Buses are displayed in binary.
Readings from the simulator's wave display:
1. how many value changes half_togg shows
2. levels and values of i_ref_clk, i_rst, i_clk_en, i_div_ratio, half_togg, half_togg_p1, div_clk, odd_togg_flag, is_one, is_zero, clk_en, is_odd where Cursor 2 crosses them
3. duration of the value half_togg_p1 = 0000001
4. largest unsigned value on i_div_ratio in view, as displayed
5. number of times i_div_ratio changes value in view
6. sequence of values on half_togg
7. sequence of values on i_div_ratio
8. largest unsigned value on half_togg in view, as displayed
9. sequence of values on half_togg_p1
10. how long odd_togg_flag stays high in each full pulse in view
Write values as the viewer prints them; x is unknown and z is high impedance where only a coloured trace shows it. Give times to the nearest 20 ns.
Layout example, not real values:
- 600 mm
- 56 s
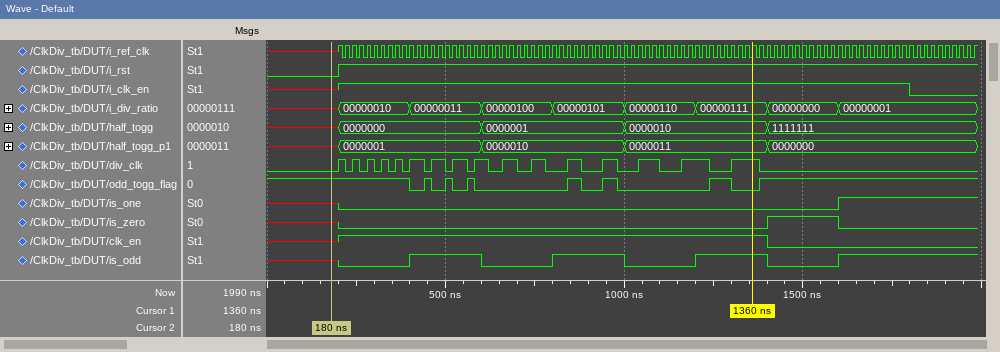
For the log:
- 4
- i_ref_clk=x, i_rst=0, i_clk_en=x, i_div_ratio=x, half_togg=x, half_togg_p1=x, div_clk=0, odd_togg_flag=1, is_one=x, is_zero=x, clk_en=x, is_odd=x
- 400 ns
- 00000111
- 8
- x, 0000000, 0000001, 0000010, 1111111
- x, 00000010, 00000011, 00000100, 00000101, 00000110, 00000111, 00000000, 00000001
- 1111111
- x, 0000001, 0000010, 0000011, 0000000
- 20 ns, 20 ns, 20 ns, 40 ns, 40 ns, 60 ns
